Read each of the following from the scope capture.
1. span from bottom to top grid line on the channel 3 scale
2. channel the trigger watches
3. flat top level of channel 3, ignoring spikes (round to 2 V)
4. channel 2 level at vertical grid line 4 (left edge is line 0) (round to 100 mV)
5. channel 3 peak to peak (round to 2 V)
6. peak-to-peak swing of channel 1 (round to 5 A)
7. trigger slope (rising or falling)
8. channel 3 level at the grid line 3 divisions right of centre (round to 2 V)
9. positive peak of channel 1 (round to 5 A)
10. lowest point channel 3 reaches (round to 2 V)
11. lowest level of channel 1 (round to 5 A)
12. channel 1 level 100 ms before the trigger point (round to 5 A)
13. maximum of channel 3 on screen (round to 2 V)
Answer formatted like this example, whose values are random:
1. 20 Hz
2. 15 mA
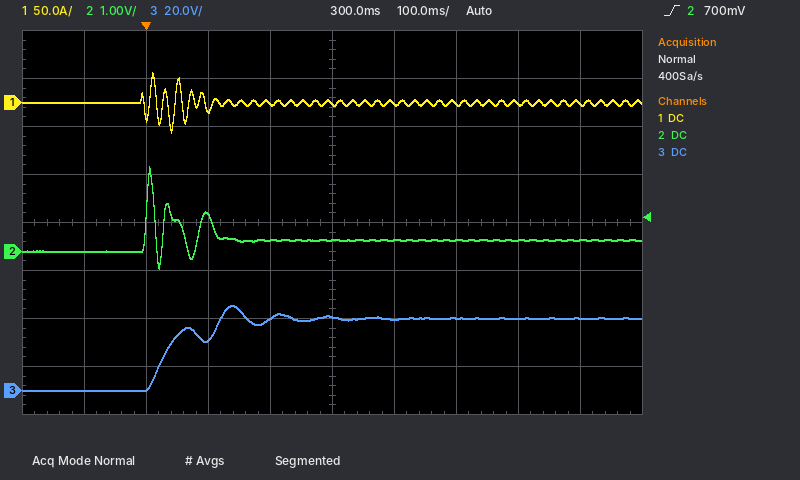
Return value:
1. 160 V
2. channel 2
3. 30 V
4. 200 mV
5. 36 V
6. 60 A
7. rising
8. 30 V
9. 30 A
10. 0 V
11. -30 A
12. 0 A
13. 36 V
